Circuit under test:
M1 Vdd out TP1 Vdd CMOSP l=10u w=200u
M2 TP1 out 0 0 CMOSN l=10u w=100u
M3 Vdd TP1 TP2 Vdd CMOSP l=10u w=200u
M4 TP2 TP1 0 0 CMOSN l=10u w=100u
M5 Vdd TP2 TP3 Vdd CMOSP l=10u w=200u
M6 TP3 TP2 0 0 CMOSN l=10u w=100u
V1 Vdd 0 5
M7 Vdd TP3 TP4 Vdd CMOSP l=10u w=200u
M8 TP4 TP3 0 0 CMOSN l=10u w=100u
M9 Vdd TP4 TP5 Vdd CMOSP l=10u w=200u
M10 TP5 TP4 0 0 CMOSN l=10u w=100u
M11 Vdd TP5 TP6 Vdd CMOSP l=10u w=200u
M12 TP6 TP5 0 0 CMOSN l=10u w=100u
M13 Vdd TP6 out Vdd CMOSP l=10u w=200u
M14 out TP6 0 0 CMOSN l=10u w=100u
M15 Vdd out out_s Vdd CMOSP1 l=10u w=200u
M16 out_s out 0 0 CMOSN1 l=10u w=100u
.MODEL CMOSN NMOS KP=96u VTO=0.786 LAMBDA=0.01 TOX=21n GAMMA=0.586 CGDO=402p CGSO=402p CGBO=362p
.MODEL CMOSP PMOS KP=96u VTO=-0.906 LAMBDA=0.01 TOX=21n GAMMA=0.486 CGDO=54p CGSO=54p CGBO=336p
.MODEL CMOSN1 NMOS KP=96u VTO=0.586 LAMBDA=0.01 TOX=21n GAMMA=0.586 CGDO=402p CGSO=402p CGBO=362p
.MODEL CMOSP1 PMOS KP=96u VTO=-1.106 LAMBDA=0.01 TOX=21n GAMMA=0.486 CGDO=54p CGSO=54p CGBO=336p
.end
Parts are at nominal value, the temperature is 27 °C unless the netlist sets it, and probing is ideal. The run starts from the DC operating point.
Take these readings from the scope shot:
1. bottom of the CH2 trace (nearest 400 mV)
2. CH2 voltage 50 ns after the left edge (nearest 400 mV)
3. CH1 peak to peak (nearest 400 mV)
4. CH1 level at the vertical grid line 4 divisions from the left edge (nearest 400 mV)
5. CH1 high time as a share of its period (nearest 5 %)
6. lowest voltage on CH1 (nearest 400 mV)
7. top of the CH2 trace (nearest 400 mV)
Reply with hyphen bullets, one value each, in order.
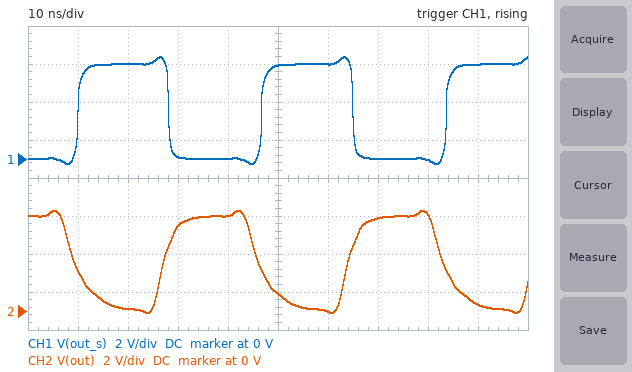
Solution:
- 0 V
- 800 mV
- 5.6 V
- 0 V
- 50 %
- -400 mV
- 5.2 V
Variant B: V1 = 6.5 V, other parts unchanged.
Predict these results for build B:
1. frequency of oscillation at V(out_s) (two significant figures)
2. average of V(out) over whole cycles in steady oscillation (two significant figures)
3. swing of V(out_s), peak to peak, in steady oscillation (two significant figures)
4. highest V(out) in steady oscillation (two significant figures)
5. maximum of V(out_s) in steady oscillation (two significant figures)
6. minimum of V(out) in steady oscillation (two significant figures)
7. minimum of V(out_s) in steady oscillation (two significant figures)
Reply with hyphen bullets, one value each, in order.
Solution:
- 39 MHz
- 3.5 V
- 7.3 V
- 6.8 V
- 6.9 V
- -110 mV
- -330 mV
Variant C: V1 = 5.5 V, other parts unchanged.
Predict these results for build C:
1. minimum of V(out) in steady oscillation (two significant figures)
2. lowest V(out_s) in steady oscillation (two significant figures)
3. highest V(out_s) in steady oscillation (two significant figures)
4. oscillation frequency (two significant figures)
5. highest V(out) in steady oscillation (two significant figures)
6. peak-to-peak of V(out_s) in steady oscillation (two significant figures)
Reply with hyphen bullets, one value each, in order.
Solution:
- -100 mV
- -280 mV
- 5.9 V
- 31 MHz
- 5.8 V
- 6.2 V
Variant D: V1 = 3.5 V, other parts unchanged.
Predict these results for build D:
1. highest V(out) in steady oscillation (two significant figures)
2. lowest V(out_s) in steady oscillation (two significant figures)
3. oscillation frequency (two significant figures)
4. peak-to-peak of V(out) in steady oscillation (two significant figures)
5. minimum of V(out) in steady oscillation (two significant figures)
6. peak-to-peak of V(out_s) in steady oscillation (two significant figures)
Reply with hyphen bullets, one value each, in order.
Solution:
- 3.7 V
- -200 mV
- 16 MHz
- 3.8 V
- -96 mV
- 4.0 V
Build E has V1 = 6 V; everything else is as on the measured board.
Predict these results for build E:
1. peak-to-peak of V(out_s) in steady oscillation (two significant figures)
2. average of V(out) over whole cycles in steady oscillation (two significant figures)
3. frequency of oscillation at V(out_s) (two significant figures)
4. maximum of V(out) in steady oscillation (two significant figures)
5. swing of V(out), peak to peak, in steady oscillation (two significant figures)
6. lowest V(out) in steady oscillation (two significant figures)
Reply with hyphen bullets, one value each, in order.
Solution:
- 6.7 V
- 3.2 V
- 35 MHz
- 6.3 V
- 6.4 V
- -110 mV
